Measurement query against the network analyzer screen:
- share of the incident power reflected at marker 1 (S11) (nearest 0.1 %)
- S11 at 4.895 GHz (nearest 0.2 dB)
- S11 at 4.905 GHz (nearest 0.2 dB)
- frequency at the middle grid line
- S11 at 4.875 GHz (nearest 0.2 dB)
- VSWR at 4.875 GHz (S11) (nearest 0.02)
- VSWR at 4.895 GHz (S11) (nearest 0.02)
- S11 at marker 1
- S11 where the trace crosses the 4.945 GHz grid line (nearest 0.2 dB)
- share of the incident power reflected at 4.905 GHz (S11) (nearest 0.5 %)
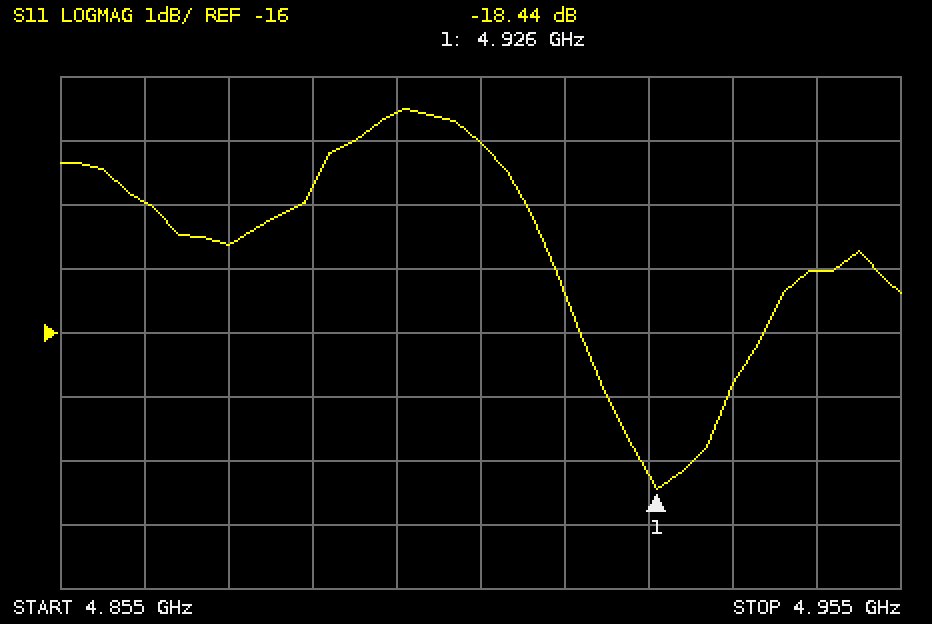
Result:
1.4 %
-12.6 dB
-13.0 dB
4.905 GHz
-14.6 dB
1.46
1.62
-18.44 dB
-15.0 dB
5.0 %
